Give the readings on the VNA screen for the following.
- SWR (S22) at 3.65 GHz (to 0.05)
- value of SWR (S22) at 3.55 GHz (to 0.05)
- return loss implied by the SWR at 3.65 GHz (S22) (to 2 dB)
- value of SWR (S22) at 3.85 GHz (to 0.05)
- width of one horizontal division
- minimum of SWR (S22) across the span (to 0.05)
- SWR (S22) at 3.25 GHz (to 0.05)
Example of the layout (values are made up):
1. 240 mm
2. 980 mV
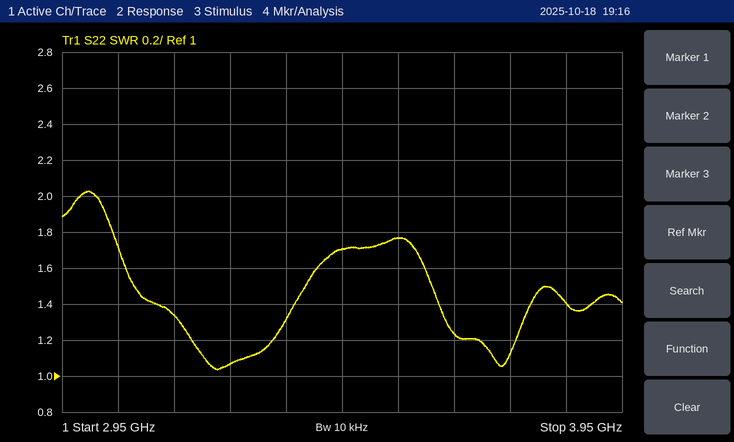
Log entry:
1. 1.25
2. 1.75
3. 20 dB
4. 1.40
5. 100 MHz
6. 1.05
7. 1.05
